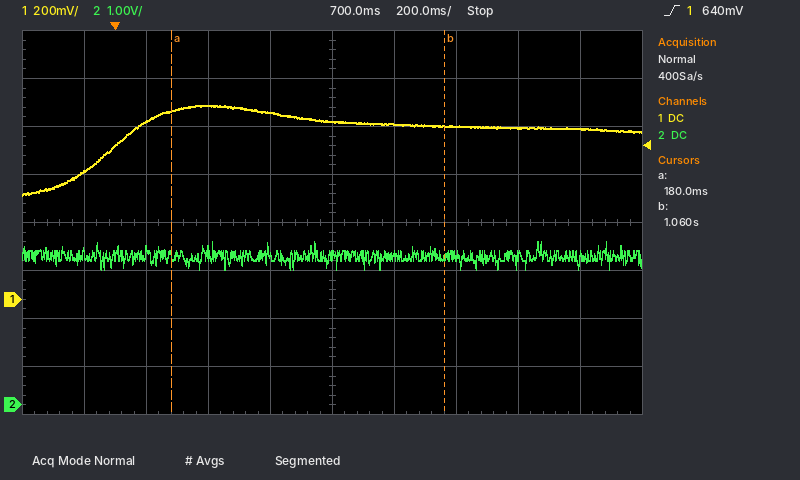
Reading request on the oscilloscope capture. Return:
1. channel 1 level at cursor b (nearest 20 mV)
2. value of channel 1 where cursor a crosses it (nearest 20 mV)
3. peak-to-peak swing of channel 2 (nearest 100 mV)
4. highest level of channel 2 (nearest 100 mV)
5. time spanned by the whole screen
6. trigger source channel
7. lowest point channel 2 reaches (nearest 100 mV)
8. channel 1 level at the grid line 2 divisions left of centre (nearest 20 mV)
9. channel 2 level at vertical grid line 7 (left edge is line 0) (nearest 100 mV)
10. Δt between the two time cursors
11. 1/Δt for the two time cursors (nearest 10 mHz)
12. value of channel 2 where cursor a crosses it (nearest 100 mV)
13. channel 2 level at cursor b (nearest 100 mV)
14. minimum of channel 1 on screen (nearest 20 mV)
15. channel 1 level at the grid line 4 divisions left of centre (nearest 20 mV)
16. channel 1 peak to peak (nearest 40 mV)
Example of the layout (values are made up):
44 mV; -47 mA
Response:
720 mV; 780 mV; 600 mV; 3.4 V; 2 s; channel 1; 2.8 V; 800 mV; 3.1 V; 880 ms; 1.14 Hz; 3.1 V; 3.1 V; 440 mV; 540 mV; 360 mV
